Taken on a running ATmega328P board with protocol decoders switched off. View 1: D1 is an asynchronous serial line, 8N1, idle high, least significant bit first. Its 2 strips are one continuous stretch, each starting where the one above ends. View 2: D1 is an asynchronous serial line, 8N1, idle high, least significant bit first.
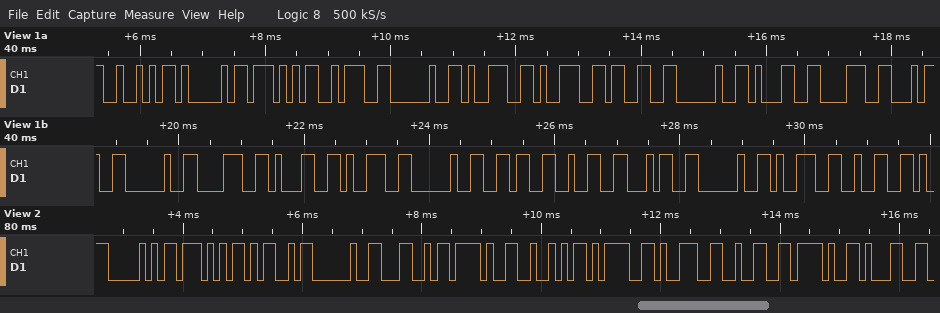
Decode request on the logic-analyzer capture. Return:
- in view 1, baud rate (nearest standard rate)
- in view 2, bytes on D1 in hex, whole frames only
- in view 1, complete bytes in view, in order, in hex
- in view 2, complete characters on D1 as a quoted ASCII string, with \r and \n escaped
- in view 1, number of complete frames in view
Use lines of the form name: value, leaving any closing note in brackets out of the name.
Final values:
in view 1, baud rate: 9600 baud
in view 2, bytes on D1 in hex, whole frames only: 50 57 4D 20 4C 2F 52 3D 39 32 2F 31
in view 1, complete bytes in view, in order, in hex: 52 41 57 3A 20 39 39 33 20 31 38 34 20 38 31 39 20 36 32 34 20 39 32
in view 2, complete characters on D1 as a quoted ASCII string, with \r and \n escaped: "PWM L/R=92/1"
in view 1, number of complete frames in view: 23
